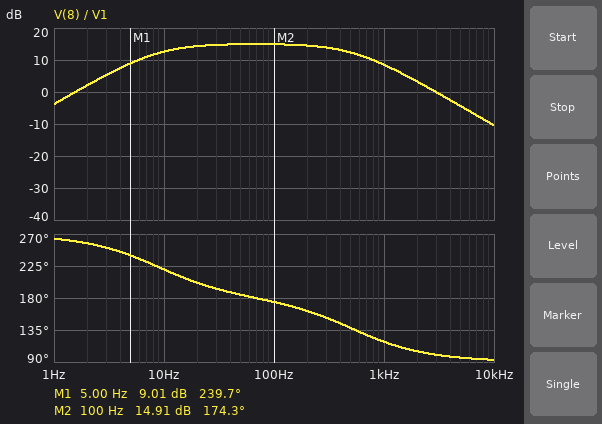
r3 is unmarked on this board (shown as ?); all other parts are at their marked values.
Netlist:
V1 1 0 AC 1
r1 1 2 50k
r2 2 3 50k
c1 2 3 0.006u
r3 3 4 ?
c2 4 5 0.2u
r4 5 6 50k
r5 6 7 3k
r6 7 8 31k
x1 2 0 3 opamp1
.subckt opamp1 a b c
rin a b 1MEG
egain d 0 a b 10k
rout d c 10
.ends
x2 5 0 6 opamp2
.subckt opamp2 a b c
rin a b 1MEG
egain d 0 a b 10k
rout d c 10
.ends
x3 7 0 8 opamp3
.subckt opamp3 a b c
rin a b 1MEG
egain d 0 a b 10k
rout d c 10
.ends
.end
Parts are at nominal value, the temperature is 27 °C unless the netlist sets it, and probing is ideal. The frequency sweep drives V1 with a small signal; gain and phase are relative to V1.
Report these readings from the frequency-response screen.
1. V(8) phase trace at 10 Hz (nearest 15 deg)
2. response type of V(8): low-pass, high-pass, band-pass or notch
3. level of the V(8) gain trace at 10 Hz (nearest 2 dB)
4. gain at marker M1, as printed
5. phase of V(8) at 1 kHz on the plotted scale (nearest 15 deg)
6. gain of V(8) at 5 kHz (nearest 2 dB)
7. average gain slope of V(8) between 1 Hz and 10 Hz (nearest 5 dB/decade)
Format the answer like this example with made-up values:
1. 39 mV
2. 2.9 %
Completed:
1. 225 deg
2. band-pass
3. 12 dB
4. 9.01 dB
5. 120 deg
6. -4 dB
7. 15 dB/decade
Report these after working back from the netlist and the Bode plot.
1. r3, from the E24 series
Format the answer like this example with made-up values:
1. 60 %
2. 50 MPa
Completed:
1. 91 kΩ
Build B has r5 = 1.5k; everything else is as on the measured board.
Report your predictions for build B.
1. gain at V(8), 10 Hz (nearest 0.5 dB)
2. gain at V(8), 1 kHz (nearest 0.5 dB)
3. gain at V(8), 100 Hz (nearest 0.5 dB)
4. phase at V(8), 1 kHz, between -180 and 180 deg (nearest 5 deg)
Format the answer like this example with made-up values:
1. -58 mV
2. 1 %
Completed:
1. 18.5 dB
2. 14.5 dB
3. 21.0 dB
4. 120 deg
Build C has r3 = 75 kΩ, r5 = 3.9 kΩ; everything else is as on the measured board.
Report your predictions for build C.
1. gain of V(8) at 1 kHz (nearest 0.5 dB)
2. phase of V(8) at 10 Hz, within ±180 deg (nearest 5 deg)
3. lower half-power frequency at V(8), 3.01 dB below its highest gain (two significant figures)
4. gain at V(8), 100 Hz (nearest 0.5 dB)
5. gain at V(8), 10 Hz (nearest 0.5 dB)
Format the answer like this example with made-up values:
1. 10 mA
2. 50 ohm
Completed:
1. 8.0 dB
2. -135 deg
3. 10 Hz
4. 14.5 dB
5. 11.0 dB
